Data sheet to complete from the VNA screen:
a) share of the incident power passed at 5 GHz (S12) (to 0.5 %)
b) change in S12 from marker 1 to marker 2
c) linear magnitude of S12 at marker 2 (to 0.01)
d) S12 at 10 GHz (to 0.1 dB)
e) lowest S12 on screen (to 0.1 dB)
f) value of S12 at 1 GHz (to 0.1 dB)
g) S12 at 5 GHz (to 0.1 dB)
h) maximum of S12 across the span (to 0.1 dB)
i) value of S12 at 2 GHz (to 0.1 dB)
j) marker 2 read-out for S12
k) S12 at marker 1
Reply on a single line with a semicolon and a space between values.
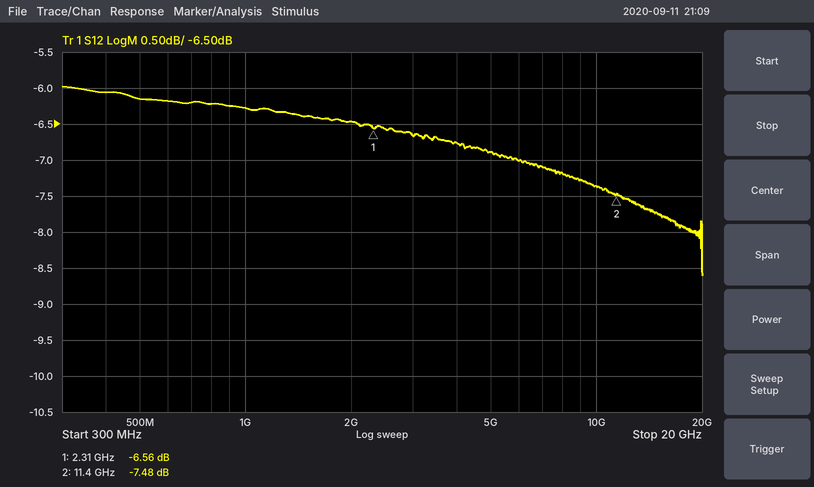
20.5 %; -0.92 dB; 0.42; -7.4 dB; -8.6 dB; -6.3 dB; -6.9 dB; -6.0 dB; -6.5 dB; -7.48 dB; -6.56 dB
